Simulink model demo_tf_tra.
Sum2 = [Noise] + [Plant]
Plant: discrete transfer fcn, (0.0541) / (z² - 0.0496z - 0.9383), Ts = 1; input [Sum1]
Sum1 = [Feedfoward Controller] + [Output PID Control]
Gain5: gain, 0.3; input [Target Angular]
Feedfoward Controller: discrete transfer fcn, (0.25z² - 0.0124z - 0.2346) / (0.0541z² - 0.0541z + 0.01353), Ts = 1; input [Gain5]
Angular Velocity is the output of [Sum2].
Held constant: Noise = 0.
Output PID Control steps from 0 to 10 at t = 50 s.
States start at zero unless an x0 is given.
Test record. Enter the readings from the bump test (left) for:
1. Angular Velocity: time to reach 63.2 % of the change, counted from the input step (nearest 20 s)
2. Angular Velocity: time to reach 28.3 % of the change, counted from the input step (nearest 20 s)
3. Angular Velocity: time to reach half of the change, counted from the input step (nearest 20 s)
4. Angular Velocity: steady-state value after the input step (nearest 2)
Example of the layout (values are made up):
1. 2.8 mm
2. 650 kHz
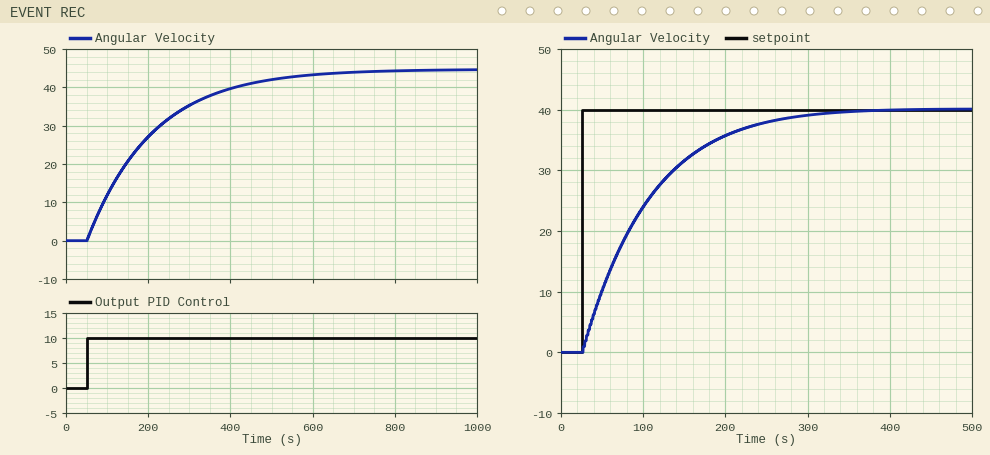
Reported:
1. 160 s
2. 60 s
3. 120 s
4. 44
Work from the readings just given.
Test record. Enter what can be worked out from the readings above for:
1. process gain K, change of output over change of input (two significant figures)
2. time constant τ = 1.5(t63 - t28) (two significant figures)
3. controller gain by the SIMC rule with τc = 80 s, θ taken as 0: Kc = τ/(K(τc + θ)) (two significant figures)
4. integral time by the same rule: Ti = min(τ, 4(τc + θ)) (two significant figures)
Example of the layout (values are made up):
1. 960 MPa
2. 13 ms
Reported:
1. 4.4
2. 150 s
3. 0.43
4. 150 s
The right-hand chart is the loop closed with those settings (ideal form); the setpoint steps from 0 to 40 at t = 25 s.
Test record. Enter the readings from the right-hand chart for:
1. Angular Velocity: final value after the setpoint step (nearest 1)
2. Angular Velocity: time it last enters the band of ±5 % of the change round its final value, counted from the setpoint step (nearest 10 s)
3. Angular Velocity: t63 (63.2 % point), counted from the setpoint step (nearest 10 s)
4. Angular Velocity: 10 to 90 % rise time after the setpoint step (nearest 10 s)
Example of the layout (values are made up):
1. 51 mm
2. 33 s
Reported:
1. 40
2. 230 s
3. 80 s
4. 170 s
